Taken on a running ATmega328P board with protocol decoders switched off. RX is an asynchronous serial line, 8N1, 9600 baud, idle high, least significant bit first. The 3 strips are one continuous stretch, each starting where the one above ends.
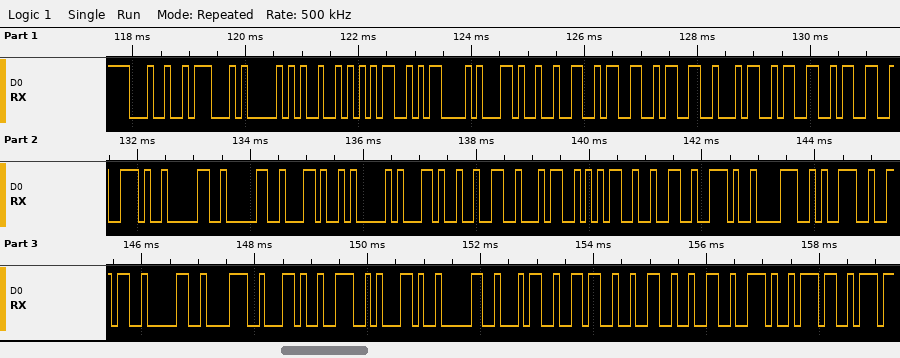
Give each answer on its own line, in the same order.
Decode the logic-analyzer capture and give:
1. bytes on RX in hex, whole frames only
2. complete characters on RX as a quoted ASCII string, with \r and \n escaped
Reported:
0x24 0x47 0x50 0x52 0x4D 0x43 0x2C 0x32 0x33 0x33 0x34 0x33 0x33 0x2E 0x30 0x30 0x2C 0x41 0x2C 0x32 0x34 0x35 0x32 0x2E 0x38 0x39 0x36 0x30 0x38 0x2C 0x4E 0x2C 0x30 0x34 0x36 0x32 0x32 0x2E 0x37
"$GPRMC,233433.00,A,2452.89608,N,04622.7"
